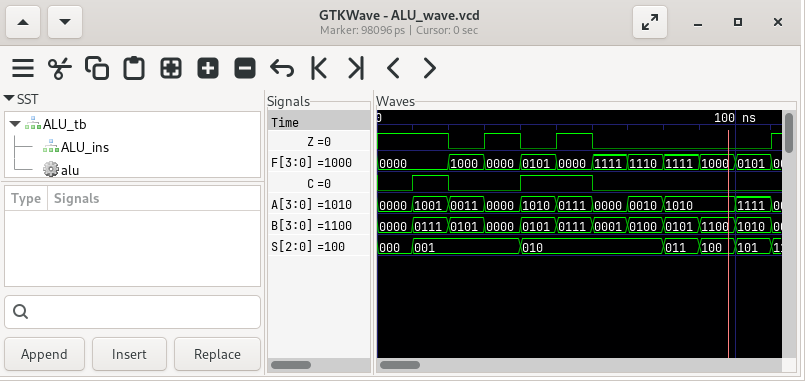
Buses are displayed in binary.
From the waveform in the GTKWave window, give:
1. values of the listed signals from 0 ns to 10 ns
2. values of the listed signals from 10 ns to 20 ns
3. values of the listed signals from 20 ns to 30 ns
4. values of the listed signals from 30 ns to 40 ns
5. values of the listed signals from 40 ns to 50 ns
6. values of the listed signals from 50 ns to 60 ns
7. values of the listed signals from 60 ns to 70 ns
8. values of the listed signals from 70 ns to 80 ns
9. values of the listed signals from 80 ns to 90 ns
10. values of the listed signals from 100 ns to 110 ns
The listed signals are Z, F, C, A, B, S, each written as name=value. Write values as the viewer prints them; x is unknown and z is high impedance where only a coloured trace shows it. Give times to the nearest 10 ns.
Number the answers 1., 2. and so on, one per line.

1. Z=1, F=0000, C=0, A=0000, B=0000, S=000
2. Z=1, F=0000, C=1, A=1001, B=0111, S=001
3. Z=0, F=1000, C=0, A=0011, B=0101, S=001
4. Z=1, F=0000, C=0, A=0000, B=0000, S=001
5. Z=0, F=0101, C=1, A=1010, B=0101, S=010
6. Z=1, F=0000, C=1, A=0111, B=0111, S=010
7. Z=0, F=1111, C=0, A=0000, B=0001, S=010
8. Z=0, F=1110, C=0, A=0010, B=0100, S=010
9. Z=0, F=1111, C=0, A=1010, B=0101, S=011
10. Z=0, F=0101, C=0, A=1111, B=1010, S=101
